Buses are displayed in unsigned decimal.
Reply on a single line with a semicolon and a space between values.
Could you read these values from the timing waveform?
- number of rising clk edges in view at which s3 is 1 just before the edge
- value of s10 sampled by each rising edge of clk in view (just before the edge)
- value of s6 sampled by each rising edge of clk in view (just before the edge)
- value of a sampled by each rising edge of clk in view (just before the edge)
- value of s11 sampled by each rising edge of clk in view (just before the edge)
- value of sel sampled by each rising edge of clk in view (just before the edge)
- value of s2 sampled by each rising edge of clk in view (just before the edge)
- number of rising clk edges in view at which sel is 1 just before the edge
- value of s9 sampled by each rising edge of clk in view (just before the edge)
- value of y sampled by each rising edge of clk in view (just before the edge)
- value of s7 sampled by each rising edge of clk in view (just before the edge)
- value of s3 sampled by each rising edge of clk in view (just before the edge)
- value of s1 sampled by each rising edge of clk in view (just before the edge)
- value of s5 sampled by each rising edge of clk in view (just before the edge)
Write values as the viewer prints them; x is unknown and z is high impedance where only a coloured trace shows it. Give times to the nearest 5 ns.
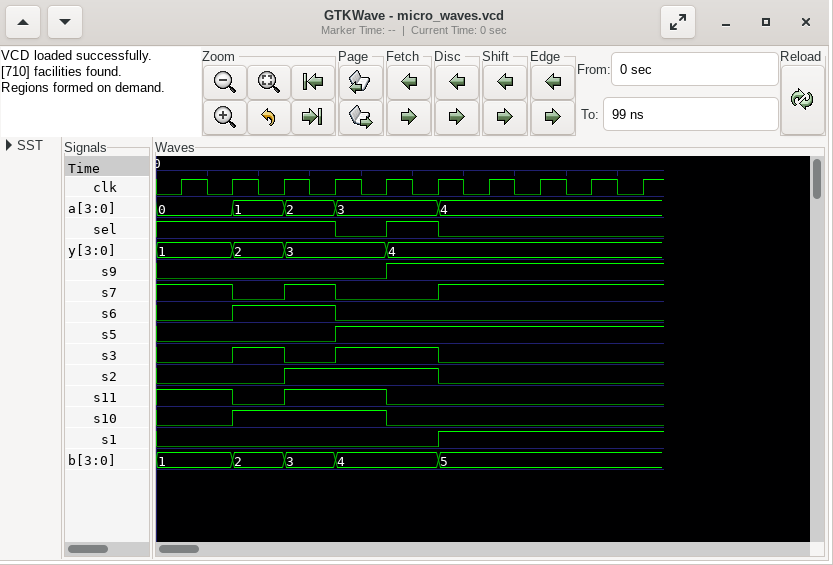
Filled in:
3; 0 0 1 1 1 0 0 0 0 0; 0 0 1 1 0 0 0 0 0 0; 0, 0, 1, 2, 3, 3, 4, 4, 4, 4; 1 1 0 1 1 0 0 0 0 0; 1 1 1 1 0 1 0 0 0 0; 0 0 0 1 1 1 0 0 0 0; 5; 0 0 0 0 0 1 1 1 1 1; 1, 1, 2, 3, 3, 4, 4, 4, 4, 4; 1 1 0 1 0 0 1 1 1 1; 0 0 1 0 1 1 0 0 0 0; 0 0 0 0 0 0 1 1 1 1; 0 0 0 0 1 1 1 1 1 1
